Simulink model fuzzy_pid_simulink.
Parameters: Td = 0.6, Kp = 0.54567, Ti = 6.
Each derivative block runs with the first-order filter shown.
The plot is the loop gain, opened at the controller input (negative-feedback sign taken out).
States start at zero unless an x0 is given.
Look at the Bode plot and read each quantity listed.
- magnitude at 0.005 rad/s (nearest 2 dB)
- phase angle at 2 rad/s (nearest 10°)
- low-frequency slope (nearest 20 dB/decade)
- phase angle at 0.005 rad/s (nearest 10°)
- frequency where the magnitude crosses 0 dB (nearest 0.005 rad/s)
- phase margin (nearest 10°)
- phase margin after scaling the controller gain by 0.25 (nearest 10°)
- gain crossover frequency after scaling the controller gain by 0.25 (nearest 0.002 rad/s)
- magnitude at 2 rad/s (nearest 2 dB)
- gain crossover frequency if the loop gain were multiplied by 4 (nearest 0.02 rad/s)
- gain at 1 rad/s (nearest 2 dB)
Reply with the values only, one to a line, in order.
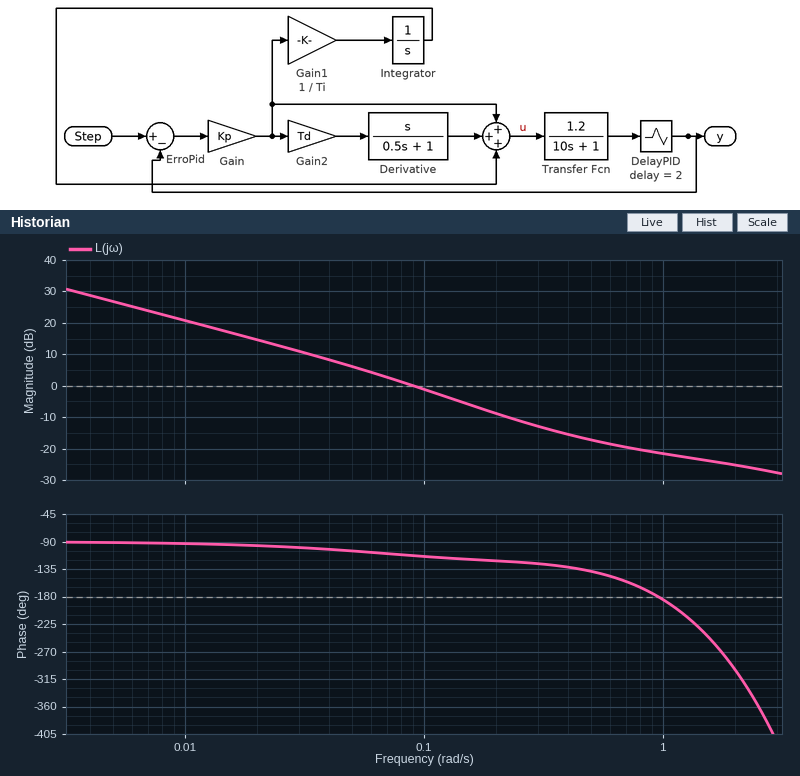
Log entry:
26 dB
-300°
-20 dB/decade
-90°
0.090 rad/s
70°
80°
0.026 rad/s
-26 dB
0.28 rad/s
-22 dB
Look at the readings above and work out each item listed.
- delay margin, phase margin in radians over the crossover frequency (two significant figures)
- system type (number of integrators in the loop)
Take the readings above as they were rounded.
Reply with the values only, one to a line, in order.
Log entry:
14 s
1
